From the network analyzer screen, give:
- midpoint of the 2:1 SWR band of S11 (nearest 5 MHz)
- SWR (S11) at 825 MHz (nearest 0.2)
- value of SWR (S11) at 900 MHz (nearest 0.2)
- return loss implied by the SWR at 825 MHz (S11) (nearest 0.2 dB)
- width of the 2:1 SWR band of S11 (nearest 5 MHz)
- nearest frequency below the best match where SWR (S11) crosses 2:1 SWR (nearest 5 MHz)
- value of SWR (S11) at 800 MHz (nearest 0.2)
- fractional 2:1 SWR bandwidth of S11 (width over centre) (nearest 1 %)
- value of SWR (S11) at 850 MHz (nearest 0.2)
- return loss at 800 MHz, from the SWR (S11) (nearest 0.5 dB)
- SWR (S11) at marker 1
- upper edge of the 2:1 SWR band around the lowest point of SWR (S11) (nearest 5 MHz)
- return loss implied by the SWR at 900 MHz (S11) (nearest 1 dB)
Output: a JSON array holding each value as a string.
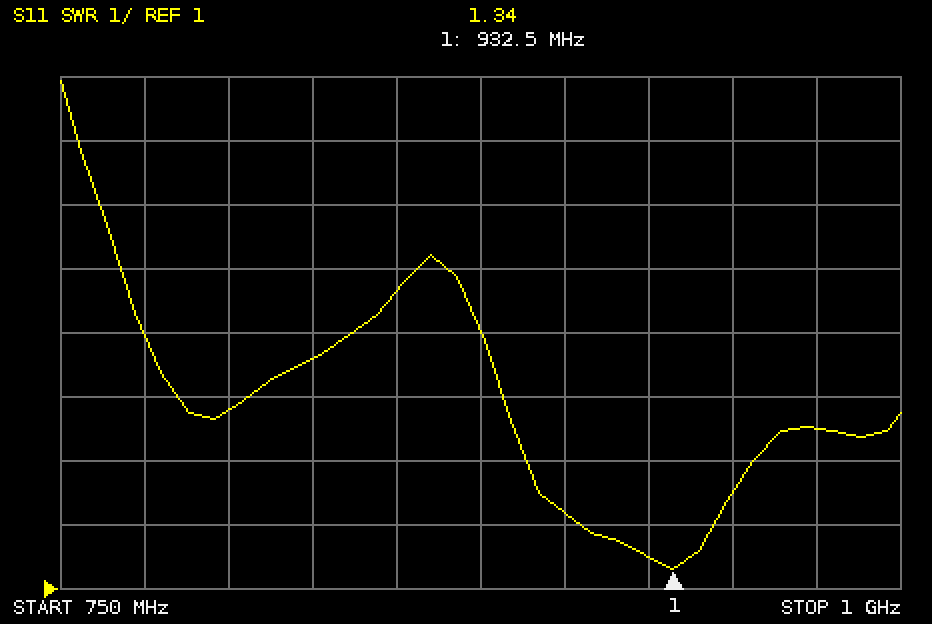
["925 MHz", "4.6", "2.2", "3.8 dB", "40 MHz", "905 MHz", "3.8", "4 %", "5.6", "4.5 dB", "1.34", "945 MHz", "9 dB"]
